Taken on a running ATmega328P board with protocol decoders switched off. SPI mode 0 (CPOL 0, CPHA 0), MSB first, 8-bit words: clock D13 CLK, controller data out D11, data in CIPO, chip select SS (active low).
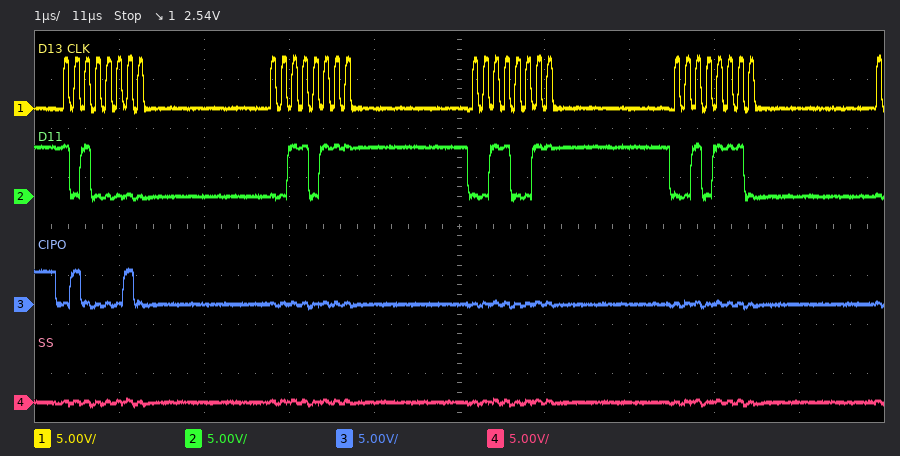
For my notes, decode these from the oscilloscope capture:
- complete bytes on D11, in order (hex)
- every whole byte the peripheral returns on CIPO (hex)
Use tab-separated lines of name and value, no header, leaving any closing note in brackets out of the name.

complete bytes on D11, in order	A0 37 33 2E
every whole byte the peripheral returns on CIPO	42 00 00 00
